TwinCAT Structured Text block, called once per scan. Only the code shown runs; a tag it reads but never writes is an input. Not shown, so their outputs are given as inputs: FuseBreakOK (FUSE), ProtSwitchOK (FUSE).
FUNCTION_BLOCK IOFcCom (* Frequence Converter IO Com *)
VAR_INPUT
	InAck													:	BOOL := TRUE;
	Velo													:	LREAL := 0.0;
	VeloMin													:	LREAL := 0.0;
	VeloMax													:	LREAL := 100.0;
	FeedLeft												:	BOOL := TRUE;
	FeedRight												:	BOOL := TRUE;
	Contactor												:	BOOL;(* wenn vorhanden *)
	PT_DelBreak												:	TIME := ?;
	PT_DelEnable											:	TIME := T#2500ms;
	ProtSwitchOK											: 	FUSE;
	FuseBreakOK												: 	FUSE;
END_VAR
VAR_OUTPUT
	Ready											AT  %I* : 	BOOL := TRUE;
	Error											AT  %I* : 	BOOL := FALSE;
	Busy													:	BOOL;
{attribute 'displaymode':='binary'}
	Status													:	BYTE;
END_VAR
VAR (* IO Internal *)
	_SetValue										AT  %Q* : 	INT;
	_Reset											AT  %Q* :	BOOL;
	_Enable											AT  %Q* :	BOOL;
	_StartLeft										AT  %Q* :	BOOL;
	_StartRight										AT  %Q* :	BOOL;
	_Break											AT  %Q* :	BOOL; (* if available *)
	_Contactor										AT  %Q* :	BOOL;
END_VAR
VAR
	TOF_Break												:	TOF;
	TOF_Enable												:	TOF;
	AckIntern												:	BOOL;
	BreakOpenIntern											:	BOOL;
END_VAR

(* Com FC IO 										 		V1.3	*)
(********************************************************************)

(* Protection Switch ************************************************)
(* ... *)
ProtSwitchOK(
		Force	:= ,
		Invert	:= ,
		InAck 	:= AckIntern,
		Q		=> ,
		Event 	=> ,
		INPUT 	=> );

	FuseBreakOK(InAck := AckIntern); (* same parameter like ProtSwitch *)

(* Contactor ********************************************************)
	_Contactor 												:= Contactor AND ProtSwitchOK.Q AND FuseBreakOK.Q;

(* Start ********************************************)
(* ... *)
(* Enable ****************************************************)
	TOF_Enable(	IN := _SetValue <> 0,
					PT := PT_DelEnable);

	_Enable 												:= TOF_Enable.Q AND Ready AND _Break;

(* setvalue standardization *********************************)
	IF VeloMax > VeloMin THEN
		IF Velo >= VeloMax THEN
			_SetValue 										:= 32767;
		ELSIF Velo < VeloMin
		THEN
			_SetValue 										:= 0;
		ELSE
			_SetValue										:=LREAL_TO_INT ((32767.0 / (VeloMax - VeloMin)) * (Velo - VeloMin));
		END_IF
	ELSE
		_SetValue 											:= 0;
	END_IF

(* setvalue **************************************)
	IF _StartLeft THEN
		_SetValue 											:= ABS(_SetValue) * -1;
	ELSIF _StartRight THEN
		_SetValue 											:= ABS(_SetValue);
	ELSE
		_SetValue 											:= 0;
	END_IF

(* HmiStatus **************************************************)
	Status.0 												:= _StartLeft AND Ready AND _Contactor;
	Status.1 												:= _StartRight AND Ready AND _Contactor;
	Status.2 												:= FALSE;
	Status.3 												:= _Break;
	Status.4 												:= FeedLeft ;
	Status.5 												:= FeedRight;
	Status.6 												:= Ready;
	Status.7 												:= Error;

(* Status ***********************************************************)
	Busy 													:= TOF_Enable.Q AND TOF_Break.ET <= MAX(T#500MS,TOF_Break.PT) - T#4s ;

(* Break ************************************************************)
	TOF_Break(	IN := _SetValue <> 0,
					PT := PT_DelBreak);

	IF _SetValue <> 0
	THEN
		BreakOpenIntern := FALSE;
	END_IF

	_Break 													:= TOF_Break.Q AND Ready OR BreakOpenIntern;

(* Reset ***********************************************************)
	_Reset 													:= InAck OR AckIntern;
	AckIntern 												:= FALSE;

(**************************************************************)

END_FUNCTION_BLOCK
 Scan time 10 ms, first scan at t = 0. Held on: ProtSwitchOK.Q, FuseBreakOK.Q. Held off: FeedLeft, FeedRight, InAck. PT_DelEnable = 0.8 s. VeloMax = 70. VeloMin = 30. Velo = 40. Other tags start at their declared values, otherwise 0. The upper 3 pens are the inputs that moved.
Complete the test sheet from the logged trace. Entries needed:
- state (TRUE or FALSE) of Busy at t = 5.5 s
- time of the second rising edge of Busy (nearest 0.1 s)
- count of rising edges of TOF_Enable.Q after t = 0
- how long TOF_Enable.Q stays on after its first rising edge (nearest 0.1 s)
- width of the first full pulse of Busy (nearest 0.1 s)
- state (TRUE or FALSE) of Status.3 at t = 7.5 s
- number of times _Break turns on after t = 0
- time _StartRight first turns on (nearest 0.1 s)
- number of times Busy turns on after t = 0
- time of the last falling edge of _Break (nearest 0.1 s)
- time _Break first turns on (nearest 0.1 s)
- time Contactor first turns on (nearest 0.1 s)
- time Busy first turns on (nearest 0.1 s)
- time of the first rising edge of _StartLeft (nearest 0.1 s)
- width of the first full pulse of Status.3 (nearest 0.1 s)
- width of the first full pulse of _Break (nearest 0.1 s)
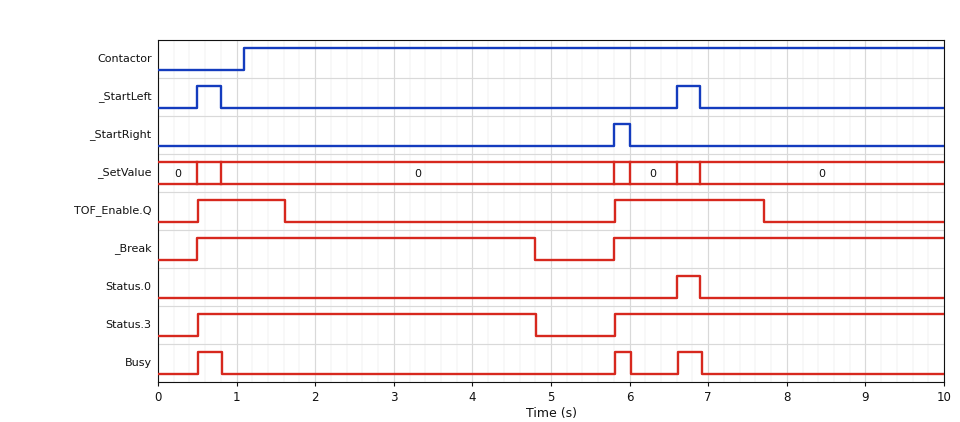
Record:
FALSE
5.8 s
2
1.1 s
0.3 s
TRUE
2
5.8 s
3
4.8 s
0.5 s
1.1 s
0.5 s
0.5 s
4.3 s
4.3 s
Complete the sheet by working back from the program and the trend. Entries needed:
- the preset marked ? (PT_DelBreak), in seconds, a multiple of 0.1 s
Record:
4.0 s
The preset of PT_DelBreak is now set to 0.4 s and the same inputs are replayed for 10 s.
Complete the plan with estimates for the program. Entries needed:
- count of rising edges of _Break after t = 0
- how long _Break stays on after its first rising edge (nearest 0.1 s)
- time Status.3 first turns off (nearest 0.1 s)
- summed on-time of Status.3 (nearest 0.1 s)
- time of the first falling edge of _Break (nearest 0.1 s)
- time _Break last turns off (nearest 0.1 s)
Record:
3
0.7 s
1.2 s
2.0 s
1.2 s
7.3 s
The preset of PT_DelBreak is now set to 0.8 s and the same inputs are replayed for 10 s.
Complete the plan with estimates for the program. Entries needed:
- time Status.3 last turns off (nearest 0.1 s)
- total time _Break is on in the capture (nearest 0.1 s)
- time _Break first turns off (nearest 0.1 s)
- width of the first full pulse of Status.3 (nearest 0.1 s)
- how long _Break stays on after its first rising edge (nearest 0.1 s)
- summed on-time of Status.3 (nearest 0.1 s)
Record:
7.7 s
3.0 s
1.6 s
1.1 s
1.1 s
3.0 s
